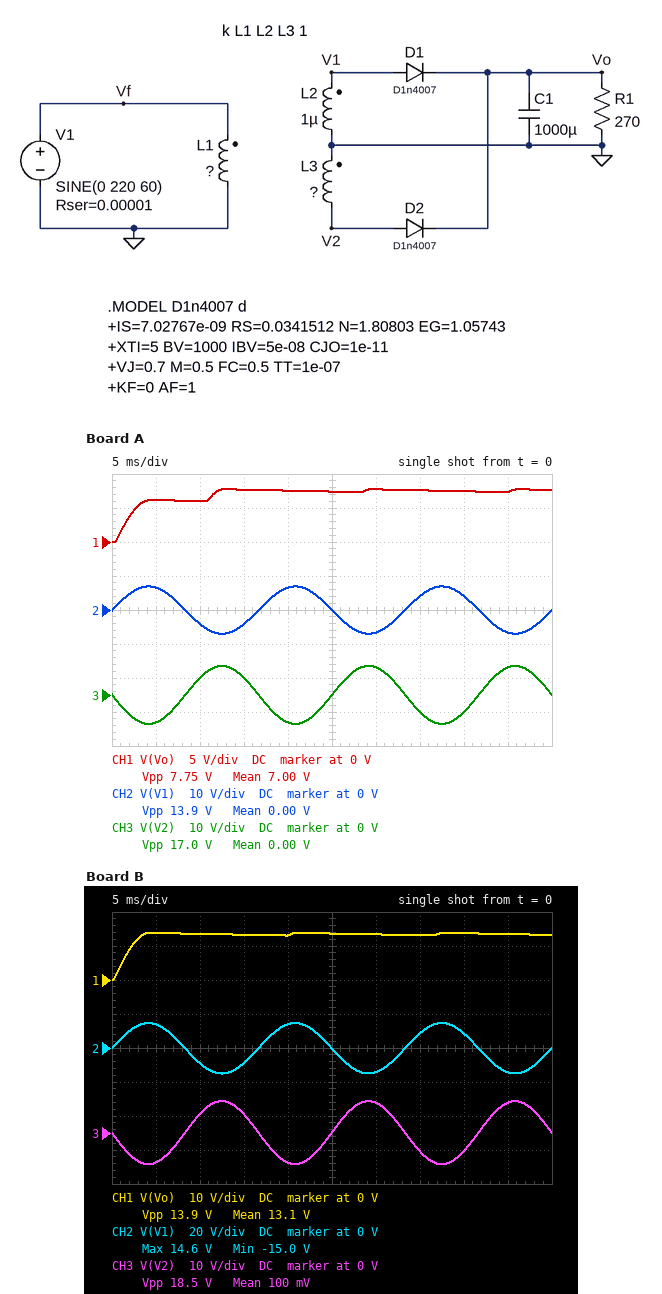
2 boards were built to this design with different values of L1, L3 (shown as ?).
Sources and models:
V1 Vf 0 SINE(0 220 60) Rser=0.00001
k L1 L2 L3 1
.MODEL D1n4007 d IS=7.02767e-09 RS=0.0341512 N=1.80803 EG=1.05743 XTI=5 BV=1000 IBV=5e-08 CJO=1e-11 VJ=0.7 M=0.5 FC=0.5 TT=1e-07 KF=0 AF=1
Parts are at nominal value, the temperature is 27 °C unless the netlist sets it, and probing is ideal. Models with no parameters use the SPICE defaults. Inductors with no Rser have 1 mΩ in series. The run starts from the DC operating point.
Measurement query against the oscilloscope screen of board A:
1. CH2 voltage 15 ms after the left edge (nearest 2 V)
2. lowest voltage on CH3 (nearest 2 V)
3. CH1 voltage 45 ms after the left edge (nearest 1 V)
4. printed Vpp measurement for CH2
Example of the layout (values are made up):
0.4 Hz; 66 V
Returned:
-4 V; -8 V; 7 V; 13.9 V
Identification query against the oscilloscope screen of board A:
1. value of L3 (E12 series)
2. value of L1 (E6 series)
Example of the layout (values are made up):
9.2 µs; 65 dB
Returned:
1.5 µH; 1 mH
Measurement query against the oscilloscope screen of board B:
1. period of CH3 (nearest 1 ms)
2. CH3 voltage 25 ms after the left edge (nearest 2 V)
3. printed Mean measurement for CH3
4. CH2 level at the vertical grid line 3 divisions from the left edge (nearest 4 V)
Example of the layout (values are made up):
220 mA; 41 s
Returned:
17 ms; 0 V; 100 mV; -8 V
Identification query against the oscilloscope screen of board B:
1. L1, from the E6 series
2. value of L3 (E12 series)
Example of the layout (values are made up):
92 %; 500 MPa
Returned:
220 µH; 390 nH
